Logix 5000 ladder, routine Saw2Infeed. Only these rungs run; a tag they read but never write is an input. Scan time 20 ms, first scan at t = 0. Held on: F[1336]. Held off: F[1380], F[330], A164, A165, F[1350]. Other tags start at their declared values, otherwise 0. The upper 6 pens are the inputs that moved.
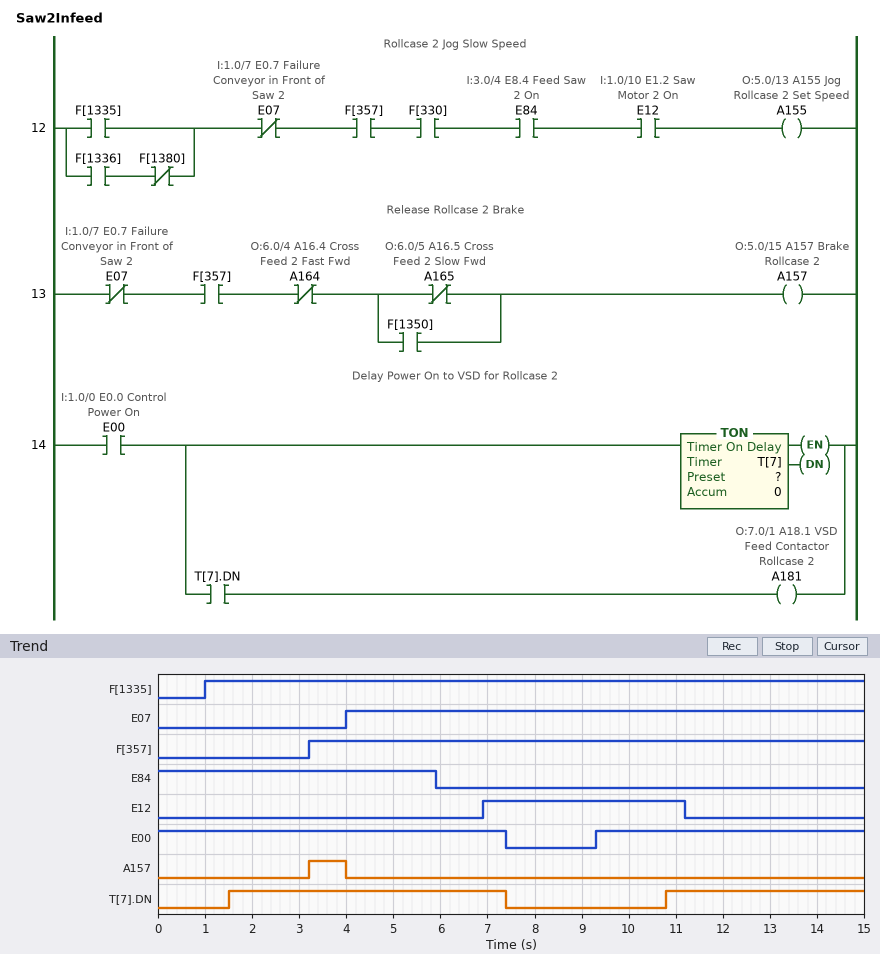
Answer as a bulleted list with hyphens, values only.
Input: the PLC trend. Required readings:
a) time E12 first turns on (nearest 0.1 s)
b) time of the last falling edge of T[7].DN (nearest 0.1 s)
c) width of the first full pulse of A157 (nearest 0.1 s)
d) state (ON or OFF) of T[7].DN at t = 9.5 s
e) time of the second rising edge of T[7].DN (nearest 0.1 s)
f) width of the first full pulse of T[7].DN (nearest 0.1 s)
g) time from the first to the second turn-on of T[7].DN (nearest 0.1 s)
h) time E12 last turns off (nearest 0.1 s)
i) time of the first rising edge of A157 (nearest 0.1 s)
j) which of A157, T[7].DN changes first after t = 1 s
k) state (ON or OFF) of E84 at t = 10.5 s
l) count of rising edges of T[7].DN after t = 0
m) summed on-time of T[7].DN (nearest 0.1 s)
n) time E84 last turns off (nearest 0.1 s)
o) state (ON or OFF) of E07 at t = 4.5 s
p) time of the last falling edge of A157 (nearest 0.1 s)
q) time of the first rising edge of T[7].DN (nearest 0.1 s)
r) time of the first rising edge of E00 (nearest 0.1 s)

- 6.9 s
- 7.4 s
- 0.8 s
- OFF
- 10.8 s
- 5.9 s
- 9.3 s
- 11.2 s
- 3.2 s
- T[7].DN
- OFF
- 2
- 10.1 s
- 5.9 s
- ON
- 4.0 s
- 1.5 s
- 9.3 s
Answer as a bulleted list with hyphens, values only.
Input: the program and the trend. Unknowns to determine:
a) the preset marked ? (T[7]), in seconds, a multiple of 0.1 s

- 1.5 s
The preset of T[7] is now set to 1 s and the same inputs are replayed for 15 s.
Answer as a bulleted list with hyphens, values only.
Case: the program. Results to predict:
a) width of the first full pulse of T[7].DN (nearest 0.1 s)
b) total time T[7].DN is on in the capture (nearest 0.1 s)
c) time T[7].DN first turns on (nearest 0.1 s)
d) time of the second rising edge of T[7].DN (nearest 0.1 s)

- 6.4 s
- 11.1 s
- 1.0 s
- 10.3 s
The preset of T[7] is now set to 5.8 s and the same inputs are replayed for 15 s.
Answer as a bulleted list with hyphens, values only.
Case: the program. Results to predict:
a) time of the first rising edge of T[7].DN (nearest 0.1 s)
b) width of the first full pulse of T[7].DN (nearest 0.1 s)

- 5.8 s
- 1.6 s
